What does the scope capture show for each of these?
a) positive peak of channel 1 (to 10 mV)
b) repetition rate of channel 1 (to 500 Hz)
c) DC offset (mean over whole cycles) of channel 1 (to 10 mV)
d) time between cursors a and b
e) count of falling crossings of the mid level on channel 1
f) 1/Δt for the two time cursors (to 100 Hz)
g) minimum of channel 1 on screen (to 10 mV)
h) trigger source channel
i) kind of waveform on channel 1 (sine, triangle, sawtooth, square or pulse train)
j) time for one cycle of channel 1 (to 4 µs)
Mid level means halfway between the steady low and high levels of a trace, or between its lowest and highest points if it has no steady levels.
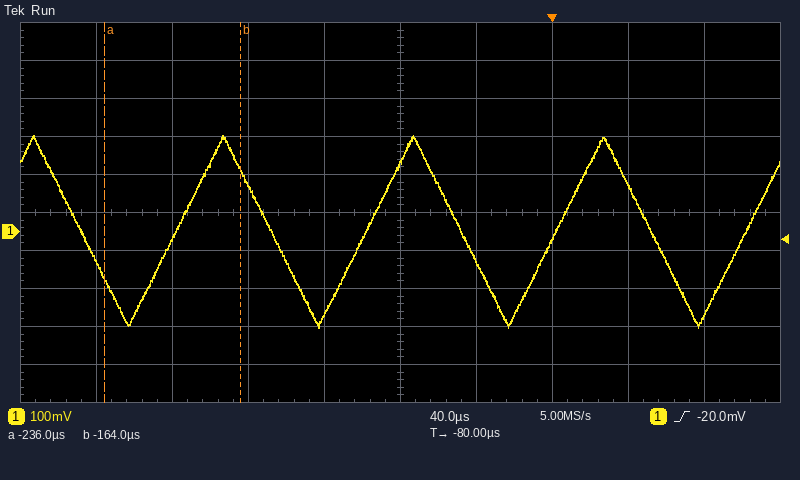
250 mV
10.0 kHz
0 mV
72 µs
4
13.9 kHz
-250 mV
channel 1
triangle
100 µs
